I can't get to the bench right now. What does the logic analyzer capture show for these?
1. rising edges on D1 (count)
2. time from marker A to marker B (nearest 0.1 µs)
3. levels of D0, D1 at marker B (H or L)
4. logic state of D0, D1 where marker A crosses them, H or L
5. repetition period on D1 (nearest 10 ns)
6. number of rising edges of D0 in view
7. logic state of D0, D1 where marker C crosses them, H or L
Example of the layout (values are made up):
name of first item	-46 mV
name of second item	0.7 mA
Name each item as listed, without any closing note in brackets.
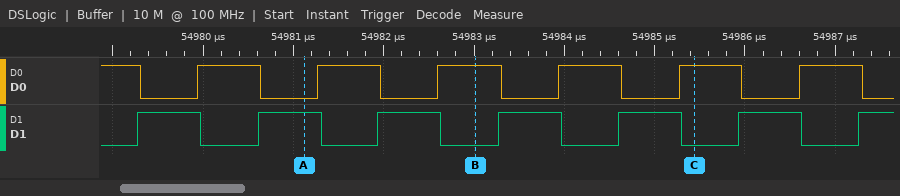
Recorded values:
rising edges on D1	7
time from marker A to marker B	1.9 µs
levels of D0, D1 at marker B	D0=H, D1=L
logic state of D0, D1 where marker A crosses them, H or L	D0=L, D1=H
repetition period on D1	1330 ns
number of rising edges of D0 in view	6
logic state of D0, D1 where marker C crosses them, H or L	D0=H, D1=L
